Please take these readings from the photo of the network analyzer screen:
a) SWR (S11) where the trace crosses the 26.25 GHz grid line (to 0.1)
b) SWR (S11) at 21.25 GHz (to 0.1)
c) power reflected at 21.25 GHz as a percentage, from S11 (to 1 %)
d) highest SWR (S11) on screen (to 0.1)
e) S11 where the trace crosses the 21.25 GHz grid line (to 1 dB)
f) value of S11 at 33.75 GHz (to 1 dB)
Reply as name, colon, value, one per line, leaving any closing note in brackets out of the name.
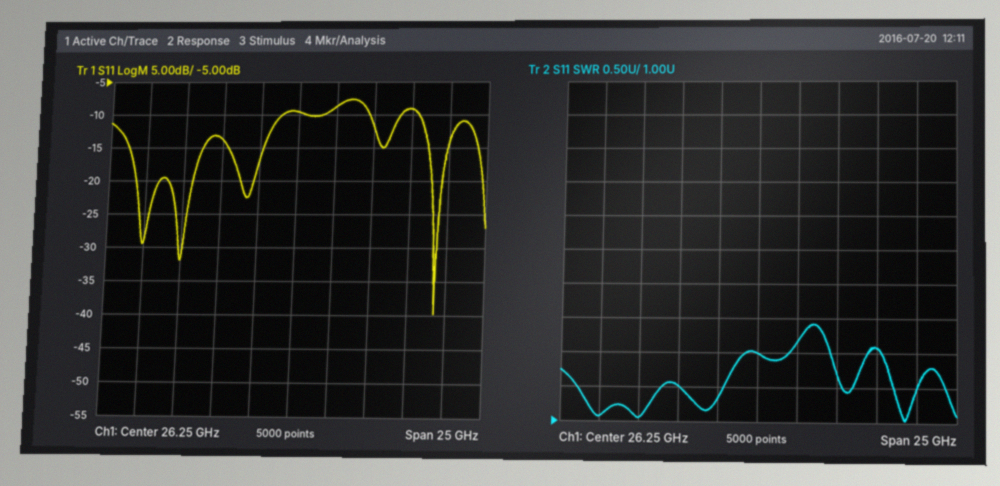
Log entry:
SWR (S11) where the trace crosses the 26.25 GHz grid line: 2.0
SWR (S11) at 21.25 GHz: 1.5
power reflected at 21.25 GHz as a percentage, from S11: 4 %
highest SWR (S11) on screen: 2.4
S11 where the trace crosses the 21.25 GHz grid line: -14 dB
value of S11 at 33.75 GHz: -9 dB
